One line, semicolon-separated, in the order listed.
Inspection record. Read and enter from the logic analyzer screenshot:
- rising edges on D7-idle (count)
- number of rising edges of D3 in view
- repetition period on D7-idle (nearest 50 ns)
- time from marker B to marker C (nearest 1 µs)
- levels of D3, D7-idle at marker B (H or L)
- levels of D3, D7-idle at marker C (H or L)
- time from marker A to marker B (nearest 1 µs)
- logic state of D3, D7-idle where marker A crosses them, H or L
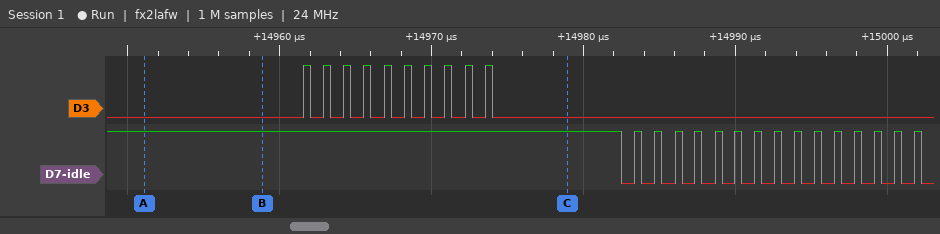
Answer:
15; 10; 1300 ns; 20 µs; D3=L, D7-idle=H; D3=L, D7-idle=H; 8 µs; D3=L, D7-idle=H
